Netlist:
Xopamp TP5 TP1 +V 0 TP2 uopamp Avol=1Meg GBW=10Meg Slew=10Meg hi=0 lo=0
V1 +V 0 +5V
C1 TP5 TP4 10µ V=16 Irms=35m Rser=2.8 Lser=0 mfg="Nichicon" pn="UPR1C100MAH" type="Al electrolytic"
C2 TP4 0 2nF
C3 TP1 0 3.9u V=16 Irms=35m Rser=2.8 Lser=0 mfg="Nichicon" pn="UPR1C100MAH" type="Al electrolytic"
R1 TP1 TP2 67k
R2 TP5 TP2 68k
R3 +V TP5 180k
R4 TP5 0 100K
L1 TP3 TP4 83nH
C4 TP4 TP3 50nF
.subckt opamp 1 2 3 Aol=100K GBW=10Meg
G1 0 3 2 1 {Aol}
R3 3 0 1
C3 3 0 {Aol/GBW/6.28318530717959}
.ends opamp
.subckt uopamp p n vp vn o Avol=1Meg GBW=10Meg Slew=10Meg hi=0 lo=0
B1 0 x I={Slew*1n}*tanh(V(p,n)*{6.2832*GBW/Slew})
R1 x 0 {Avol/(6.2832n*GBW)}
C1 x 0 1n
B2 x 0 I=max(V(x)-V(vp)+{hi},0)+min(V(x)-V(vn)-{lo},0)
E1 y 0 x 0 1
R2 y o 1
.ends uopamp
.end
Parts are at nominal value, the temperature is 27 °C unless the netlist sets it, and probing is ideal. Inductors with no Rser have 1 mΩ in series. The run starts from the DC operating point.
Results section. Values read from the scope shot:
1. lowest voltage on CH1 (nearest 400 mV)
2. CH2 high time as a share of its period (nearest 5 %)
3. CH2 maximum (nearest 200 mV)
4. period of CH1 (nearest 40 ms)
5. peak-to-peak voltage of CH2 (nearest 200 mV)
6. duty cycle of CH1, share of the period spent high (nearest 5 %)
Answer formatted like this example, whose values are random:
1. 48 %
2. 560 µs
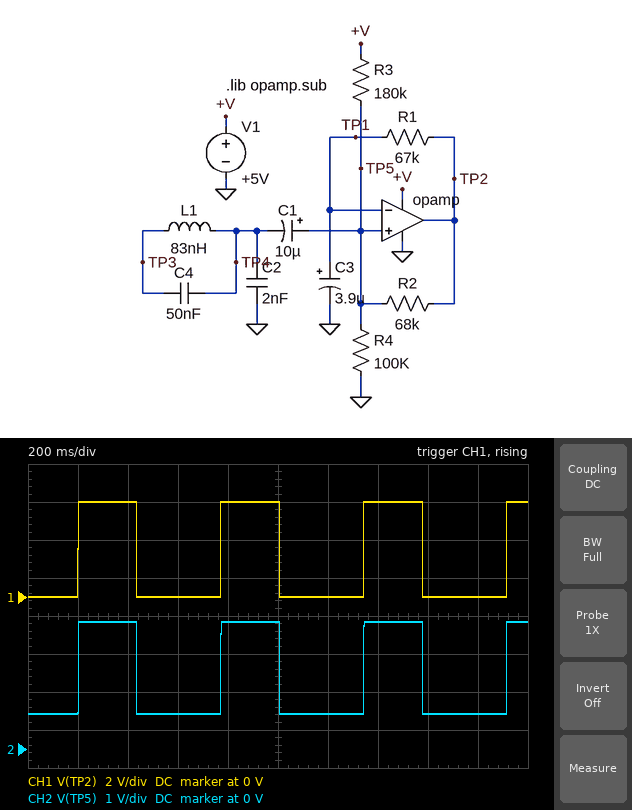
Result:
1. 0 V
2. 40 %
3. 3.4 V
4. 560 ms
5. 2.4 V
6. 40 %
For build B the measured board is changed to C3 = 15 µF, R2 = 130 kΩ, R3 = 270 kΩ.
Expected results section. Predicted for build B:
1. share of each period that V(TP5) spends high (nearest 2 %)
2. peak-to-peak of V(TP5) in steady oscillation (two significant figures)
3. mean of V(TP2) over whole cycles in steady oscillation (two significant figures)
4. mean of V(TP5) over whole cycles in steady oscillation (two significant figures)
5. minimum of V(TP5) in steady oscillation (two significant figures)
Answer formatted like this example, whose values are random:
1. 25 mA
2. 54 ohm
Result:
1. 34 %
2. 1.8 V
3. 1.7 V
4. 1.5 V
5. 860 mV
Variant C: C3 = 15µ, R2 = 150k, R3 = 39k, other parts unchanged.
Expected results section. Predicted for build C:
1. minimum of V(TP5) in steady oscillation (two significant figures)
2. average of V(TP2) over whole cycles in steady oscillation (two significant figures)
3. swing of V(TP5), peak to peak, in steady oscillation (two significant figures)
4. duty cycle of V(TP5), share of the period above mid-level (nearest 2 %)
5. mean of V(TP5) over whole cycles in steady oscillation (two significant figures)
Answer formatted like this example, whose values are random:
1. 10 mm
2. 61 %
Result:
1. 3.0 V
2. 3.4 V
3. 800 mV
4. 68 %
5. 3.6 V
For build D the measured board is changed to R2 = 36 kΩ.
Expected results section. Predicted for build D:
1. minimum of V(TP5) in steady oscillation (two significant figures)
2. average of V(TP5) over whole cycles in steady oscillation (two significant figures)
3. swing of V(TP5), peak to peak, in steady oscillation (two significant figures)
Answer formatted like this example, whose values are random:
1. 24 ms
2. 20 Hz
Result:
1. 630 mV
2. 2.0 V
3. 3.2 V
